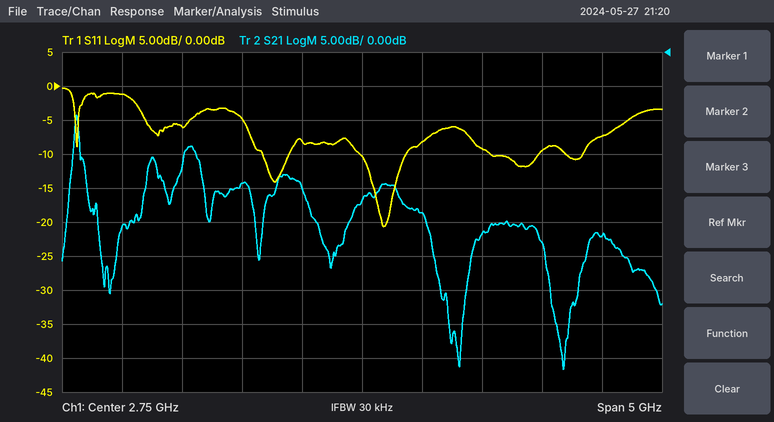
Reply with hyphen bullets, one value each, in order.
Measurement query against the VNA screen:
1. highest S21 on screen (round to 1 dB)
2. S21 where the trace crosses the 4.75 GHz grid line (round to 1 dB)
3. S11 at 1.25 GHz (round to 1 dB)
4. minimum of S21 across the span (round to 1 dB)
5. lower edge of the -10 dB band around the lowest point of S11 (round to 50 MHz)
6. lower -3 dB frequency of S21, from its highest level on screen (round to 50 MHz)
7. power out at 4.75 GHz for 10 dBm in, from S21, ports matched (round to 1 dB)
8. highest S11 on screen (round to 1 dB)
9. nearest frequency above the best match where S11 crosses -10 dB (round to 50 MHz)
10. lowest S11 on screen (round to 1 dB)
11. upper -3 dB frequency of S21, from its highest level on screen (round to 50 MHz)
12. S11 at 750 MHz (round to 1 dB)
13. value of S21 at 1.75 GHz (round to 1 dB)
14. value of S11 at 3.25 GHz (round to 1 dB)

- -9 dB
- -27 dB
- -6 dB
- -47 dB
- 2.75 GHz
- 350 MHz
- -17 dBm
- 0 dB
- 3.10 GHz
- -21 dB
- 400 MHz
- -1 dB
- -19 dB
- -8 dB
